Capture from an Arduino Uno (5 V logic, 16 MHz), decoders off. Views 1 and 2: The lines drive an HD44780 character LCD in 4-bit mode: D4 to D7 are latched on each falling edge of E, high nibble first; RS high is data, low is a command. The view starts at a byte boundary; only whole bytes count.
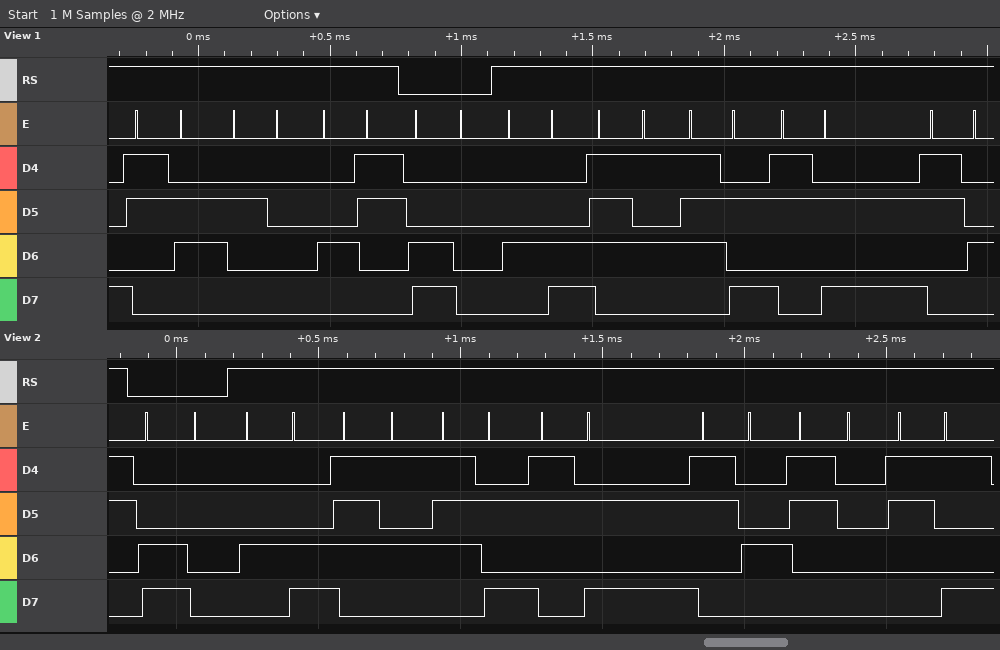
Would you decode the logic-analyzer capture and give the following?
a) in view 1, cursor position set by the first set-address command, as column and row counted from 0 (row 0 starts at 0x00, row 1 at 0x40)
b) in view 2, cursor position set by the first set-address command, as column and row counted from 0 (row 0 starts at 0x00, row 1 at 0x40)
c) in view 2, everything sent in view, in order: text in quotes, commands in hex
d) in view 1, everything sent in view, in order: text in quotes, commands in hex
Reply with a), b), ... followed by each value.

a) column 0, row 1
b) column 0, row 1
c) 0xC0 "Luz:409"
d) "6 C" 0xC0 "Luz:4"
